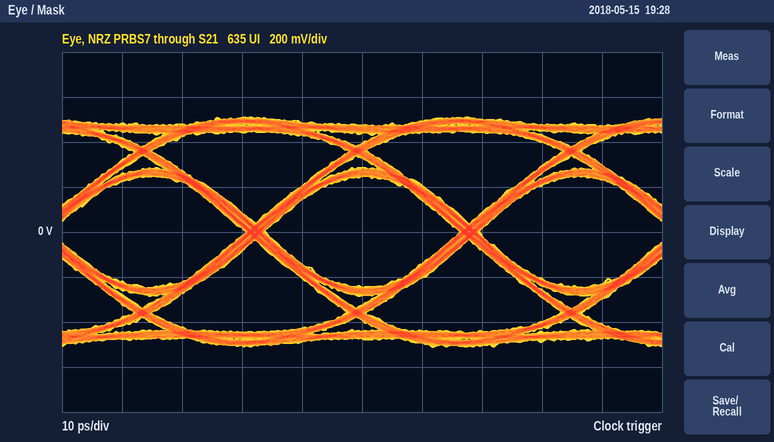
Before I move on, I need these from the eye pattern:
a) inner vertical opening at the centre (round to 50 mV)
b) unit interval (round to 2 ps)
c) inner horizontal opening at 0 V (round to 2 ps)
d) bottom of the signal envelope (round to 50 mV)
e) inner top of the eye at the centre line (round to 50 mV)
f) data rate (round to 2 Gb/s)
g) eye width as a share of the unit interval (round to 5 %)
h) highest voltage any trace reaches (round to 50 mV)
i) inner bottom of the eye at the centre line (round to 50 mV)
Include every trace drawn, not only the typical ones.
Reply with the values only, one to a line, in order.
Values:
500 mV
36 ps
32 ps
-500 mV
250 mV
28 Gb/s
90 %
500 mV
-250 mV
